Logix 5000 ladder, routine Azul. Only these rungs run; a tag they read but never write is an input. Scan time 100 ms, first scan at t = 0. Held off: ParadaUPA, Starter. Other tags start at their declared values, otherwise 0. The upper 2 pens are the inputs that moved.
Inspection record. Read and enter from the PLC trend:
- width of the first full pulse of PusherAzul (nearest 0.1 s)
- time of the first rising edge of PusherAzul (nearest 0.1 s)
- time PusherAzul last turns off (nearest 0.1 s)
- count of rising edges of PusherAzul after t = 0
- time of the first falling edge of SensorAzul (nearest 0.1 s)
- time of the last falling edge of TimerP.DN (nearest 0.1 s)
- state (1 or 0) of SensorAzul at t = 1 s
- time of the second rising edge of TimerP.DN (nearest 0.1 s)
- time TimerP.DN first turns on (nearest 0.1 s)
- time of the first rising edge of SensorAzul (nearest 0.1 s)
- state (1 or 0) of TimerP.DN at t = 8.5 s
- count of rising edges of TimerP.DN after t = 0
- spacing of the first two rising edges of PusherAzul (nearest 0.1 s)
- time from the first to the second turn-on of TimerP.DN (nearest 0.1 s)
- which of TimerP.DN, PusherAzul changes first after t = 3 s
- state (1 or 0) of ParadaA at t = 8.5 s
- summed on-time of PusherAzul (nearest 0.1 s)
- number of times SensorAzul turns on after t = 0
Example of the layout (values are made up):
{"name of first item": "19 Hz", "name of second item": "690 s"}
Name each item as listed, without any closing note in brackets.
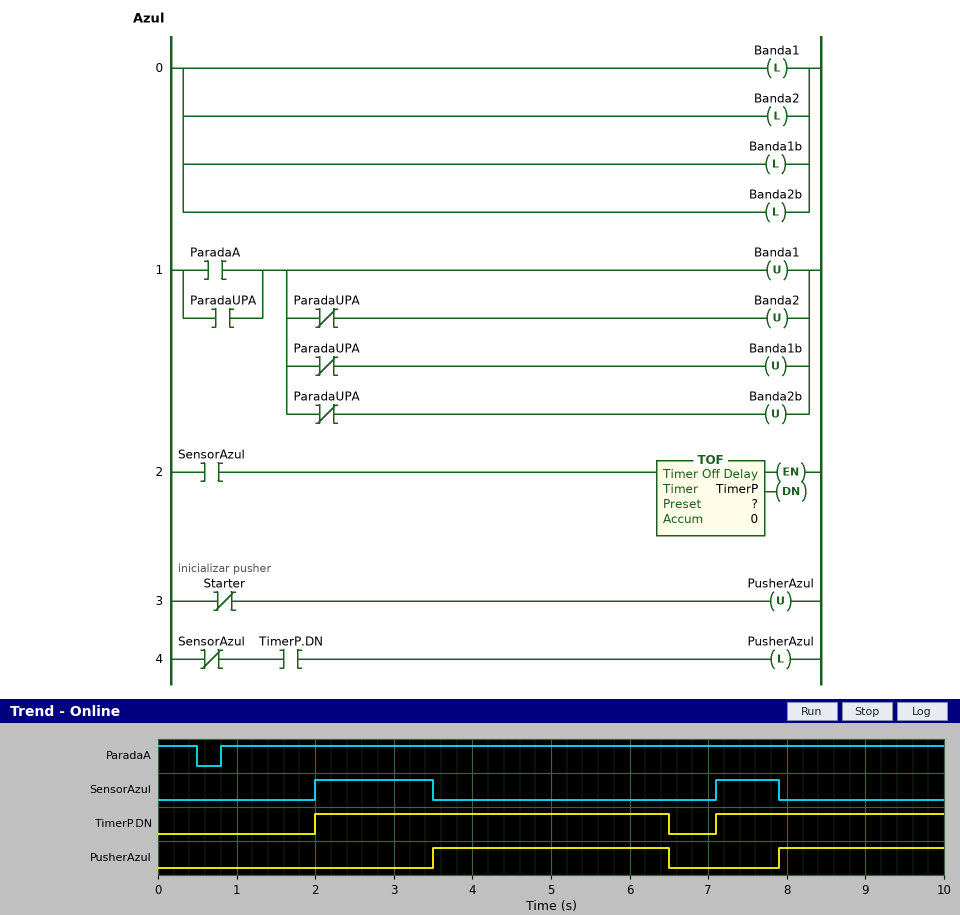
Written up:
{"width of the first full pulse of PusherAzul": "3.0 s", "time of the first rising edge of PusherAzul": "3.5 s", "time PusherAzul last turns off": "6.5 s", "count of rising edges of PusherAzul after t = 0": "2", "time of the first falling edge of SensorAzul": "3.5 s", "time of the last falling edge of TimerP.DN": "6.5 s", "state (1 or 0) of SensorAzul at t = 1 s": "0", "time of the second rising edge of TimerP.DN": "7.1 s", "time TimerP.DN first turns on": "2.0 s", "time of the first rising edge of SensorAzul": "2.0 s", "state (1 or 0) of TimerP.DN at t = 8.5 s": "1", "count of rising edges of TimerP.DN after t = 0": "2", "spacing of the first two rising edges of PusherAzul": "4.4 s", "time from the first to the second turn-on of TimerP.DN": "5.1 s", "which of TimerP.DN, PusherAzul changes first after t = 3 s": "PusherAzul", "state (1 or 0) of ParadaA at t = 8.5 s": "1", "summed on-time of PusherAzul": "5.1 s", "number of times SensorAzul turns on after t = 0": "2"}
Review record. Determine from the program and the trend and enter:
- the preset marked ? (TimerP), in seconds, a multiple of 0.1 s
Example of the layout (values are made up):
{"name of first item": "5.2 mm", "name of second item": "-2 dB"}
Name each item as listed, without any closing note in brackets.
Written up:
{"the preset marked ? (TimerP), in seconds, a multiple of 0.1 s": "3.0 s"}
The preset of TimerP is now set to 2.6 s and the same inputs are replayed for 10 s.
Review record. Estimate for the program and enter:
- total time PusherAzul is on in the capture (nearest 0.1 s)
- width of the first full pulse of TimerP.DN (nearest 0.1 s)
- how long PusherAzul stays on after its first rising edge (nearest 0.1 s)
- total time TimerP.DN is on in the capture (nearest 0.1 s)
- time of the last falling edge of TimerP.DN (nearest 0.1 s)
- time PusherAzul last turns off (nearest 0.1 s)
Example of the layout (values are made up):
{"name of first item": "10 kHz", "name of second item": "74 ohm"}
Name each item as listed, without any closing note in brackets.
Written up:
{"total time PusherAzul is on in the capture": "4.7 s", "width of the first full pulse of TimerP.DN": "4.1 s", "how long PusherAzul stays on after its first rising edge": "2.6 s", "total time TimerP.DN is on in the capture": "7.0 s", "time of the last falling edge of TimerP.DN": "6.1 s", "time PusherAzul last turns off": "6.1 s"}
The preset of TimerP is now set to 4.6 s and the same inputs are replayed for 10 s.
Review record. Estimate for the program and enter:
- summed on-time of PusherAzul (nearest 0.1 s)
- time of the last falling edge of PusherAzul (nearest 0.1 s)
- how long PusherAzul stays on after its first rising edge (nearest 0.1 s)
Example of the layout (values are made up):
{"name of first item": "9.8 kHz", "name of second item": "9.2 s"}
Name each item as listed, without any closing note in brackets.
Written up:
{"summed on-time of PusherAzul": "5.7 s", "time of the last falling edge of PusherAzul": "7.1 s", "how long PusherAzul stays on after its first rising edge": "3.6 s"}
